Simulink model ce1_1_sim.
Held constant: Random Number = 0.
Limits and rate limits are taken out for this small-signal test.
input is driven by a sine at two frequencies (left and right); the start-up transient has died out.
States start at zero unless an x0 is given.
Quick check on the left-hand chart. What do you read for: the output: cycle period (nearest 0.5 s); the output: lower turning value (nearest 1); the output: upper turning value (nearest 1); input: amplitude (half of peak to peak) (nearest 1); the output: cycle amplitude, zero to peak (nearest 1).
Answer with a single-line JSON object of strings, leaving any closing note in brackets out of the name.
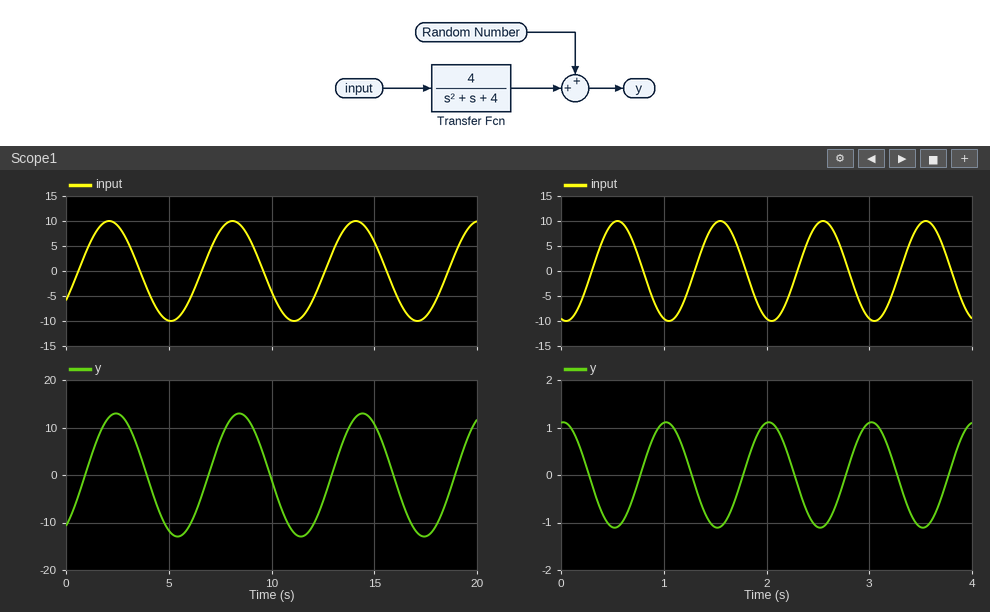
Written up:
{"the output: cycle period": "6.0 s", "the output: lower turning value": "-13", "the output: upper turning value": "13", "input: amplitude (half of peak to peak)": "10", "the output: cycle amplitude, zero to peak": "13"}
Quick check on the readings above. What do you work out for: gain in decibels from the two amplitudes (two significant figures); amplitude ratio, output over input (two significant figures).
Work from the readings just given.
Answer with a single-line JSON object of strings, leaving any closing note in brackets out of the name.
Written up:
{"gain in decibels from the two amplitudes": "2.3 dB", "amplitude ratio, output over input": "1.3"}
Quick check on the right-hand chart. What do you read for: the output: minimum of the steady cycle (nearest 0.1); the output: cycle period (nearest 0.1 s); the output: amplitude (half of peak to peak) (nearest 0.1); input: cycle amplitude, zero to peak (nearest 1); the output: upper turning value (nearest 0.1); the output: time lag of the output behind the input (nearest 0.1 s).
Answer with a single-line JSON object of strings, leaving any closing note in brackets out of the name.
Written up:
{"the output: minimum of the steady cycle": "-1.1", "the output: cycle period": "1.0 s", "the output: amplitude (half of peak to peak)": "1.1", "input: cycle amplitude, zero to peak": "10", "the output: upper turning value": "1.1", "the output: time lag of the output behind the input": "0.5 s"}
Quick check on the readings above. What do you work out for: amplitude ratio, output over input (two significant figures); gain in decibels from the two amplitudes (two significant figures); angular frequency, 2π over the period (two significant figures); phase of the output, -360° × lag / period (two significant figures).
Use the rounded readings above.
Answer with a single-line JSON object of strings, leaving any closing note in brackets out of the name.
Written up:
{"amplitude ratio, output over input": "0.11", "gain in decibels from the two amplitudes": "-19 dB", "angular frequency, 2π over the period": "6.3 rad/s", "phase of the output, -360° × lag / period": "-180°"}
